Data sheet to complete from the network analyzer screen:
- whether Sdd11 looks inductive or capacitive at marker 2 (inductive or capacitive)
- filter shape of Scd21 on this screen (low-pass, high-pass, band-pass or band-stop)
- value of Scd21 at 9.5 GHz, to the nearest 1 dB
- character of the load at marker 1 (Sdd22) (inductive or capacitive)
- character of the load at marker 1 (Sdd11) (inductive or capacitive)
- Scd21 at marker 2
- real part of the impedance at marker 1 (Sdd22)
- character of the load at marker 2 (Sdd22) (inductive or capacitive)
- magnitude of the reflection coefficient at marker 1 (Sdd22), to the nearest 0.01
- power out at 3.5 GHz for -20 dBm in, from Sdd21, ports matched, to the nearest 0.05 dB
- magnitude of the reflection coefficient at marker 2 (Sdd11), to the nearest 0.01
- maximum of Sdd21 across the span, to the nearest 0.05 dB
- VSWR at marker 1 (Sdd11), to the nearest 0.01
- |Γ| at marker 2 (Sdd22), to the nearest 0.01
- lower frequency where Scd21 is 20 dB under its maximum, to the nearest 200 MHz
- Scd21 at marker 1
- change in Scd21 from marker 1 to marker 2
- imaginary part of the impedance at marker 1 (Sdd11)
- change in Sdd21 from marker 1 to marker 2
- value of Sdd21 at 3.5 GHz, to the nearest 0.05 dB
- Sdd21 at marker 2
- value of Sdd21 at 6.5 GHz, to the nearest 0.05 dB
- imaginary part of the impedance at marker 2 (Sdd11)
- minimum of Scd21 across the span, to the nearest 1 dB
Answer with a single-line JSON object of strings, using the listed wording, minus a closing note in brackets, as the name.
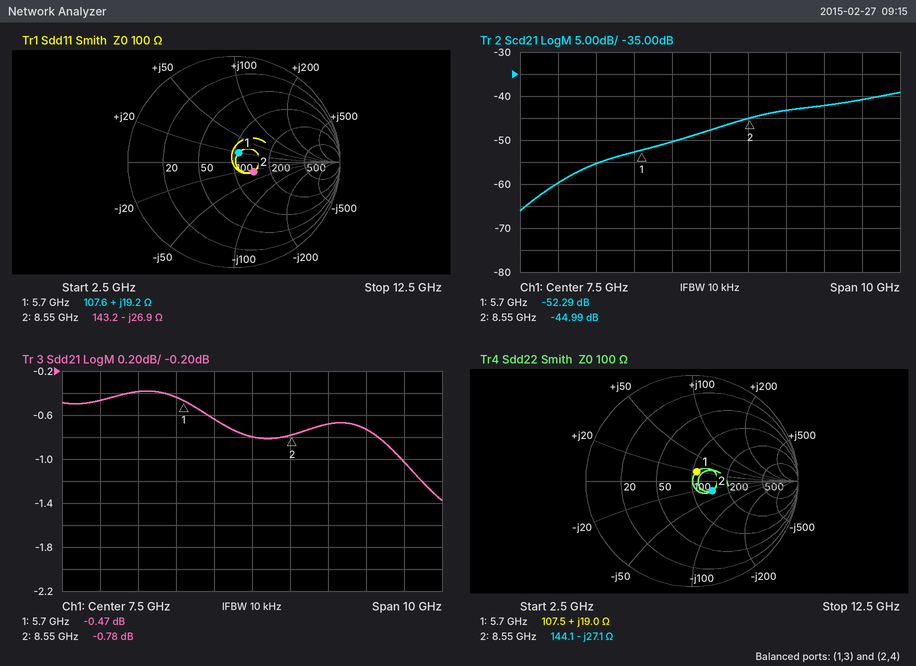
{"whether Sdd11 looks inductive or capacitive at marker 2": "capacitive", "filter shape of Scd21 on this screen": "high-pass", "value of Scd21 at 9.5 GHz, to the nearest 1 dB": "-43 dB", "character of the load at marker 1 (Sdd22)": "inductive", "character of the load at marker 1 (Sdd11)": "inductive", "Scd21 at marker 2": "-44.99 dB", "real part of the impedance at marker 1": "107.5 Ω", "character of the load at marker 2 (Sdd22)": "capacitive", "magnitude of the reflection coefficient at marker 1 (Sdd22), to the nearest 0.01": "0.10", "power out at 3.5 GHz for -20 dBm in, from Sdd21, ports matched, to the nearest 0.05 dB": "-20.45 dBm", "magnitude of the reflection coefficient at marker 2 (Sdd11), to the nearest 0.01": "0.21", "maximum of Sdd21 across the span, to the nearest 0.05 dB": "-0.40 dB", "VSWR at marker 1 (Sdd11), to the nearest 0.01": "1.22", "|Γ| at marker 2 (Sdd22), to the nearest 0.01": "0.21", "lower frequency where Scd21 is 20 dB under its maximum, to the nearest 200 MHz": "3.6 GHz", "Scd21 at marker 1": "-52.29 dB", "change in Scd21 from marker 1 to marker 2": "7.30 dB", "imaginary part of the impedance at marker 1": "+19.2 Ω", "change in Sdd21 from marker 1 to marker 2": "-0.31 dB", "value of Sdd21 at 3.5 GHz, to the nearest 0.05 dB": "-0.45 dB", "Sdd21 at marker 2": "-0.78 dB", "value of Sdd21 at 6.5 GHz, to the nearest 0.05 dB": "-0.65 dB", "imaginary part of the impedance at marker 2": "-26.9 Ω", "minimum of Scd21 across the span, to the nearest 1 dB": "-66 dB"}
